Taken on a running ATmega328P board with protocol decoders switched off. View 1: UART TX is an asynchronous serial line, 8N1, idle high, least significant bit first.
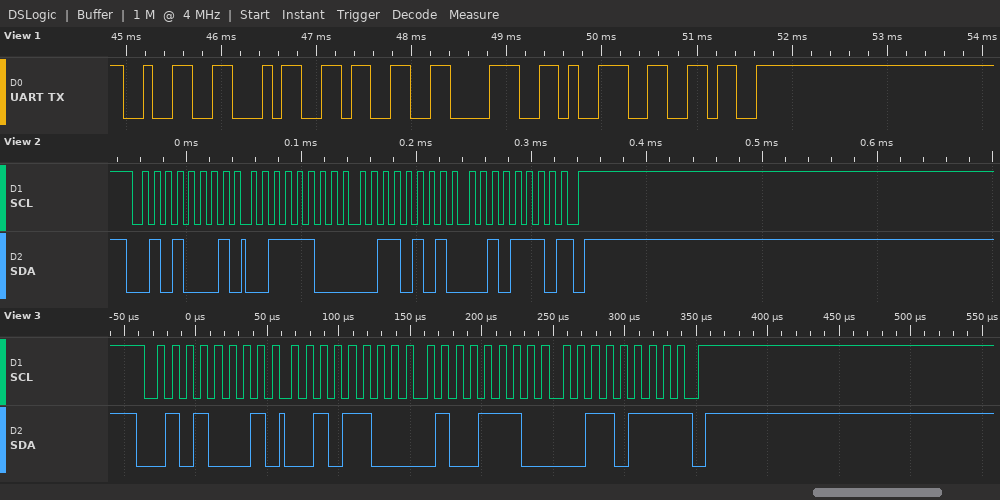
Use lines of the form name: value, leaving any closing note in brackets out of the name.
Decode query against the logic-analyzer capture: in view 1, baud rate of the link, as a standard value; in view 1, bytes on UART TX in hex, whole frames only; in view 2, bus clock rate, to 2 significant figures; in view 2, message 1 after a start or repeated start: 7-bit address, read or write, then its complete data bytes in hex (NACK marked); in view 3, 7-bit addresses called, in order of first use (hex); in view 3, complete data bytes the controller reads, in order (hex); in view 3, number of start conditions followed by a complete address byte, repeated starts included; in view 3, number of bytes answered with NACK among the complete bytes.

in view 1, baud rate of the link, as a standard value: 9600 baud
in view 1, bytes on UART TX in hex, whole frames only: 0x32 0x34 0x33 0x38 0x39 0x36
in view 2, bus clock rate, to 2 significant figures: 100 kHz
in view 2, message 1 after a start or repeated start: 7-bit address, read or write, then its complete data bytes in hex: 0x28 read: 3C 35 2E NACK
in view 3, 7-bit addresses called, in order of first use: 0x28
in view 3, complete data bytes the controller reads, in order: 2C 4E 37
in view 3, number of start conditions followed by a complete address byte, repeated starts included: 1
in view 3, number of bytes answered with NACK among the complete bytes: 1
